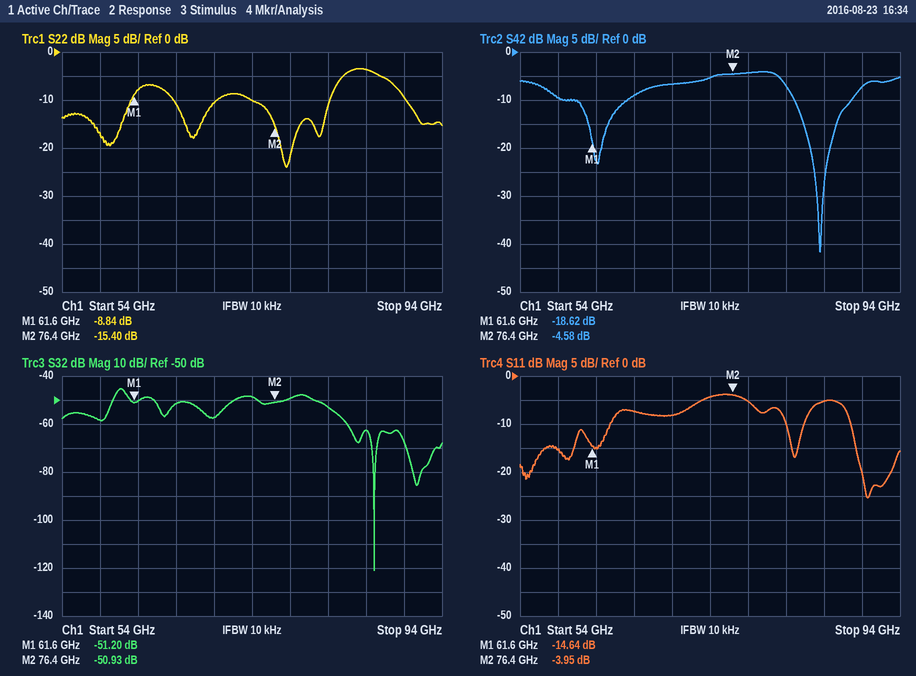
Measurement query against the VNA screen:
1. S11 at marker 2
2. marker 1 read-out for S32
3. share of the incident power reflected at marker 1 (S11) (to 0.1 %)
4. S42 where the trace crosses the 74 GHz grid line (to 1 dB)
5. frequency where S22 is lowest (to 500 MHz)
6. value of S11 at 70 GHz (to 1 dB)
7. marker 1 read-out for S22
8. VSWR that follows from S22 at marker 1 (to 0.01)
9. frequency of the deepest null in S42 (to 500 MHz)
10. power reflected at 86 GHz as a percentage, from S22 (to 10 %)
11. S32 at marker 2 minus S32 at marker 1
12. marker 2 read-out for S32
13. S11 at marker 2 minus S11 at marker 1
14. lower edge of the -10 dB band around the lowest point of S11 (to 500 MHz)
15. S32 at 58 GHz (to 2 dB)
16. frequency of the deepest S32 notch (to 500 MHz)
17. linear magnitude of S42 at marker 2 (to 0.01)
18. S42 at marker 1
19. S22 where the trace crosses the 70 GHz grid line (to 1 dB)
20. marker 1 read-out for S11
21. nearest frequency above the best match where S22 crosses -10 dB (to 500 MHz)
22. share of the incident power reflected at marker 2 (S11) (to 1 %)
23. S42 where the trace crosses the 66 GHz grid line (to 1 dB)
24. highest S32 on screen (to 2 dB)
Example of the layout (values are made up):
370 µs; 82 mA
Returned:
-3.95 dB; -51.20 dB; 3.4 %; -5 dB; 77.5 GHz; -8 dB; -8.84 dB; 2.13; 85.5 GHz; 40 %; 0.27 dB; -50.93 dB; 10.69 dB; 89.0 GHz; -58 dB; 87.0 GHz; 0.59; -18.62 dB; -11 dB; -14.64 dB; 82.0 GHz; 40 %; -9 dB; -46 dB
